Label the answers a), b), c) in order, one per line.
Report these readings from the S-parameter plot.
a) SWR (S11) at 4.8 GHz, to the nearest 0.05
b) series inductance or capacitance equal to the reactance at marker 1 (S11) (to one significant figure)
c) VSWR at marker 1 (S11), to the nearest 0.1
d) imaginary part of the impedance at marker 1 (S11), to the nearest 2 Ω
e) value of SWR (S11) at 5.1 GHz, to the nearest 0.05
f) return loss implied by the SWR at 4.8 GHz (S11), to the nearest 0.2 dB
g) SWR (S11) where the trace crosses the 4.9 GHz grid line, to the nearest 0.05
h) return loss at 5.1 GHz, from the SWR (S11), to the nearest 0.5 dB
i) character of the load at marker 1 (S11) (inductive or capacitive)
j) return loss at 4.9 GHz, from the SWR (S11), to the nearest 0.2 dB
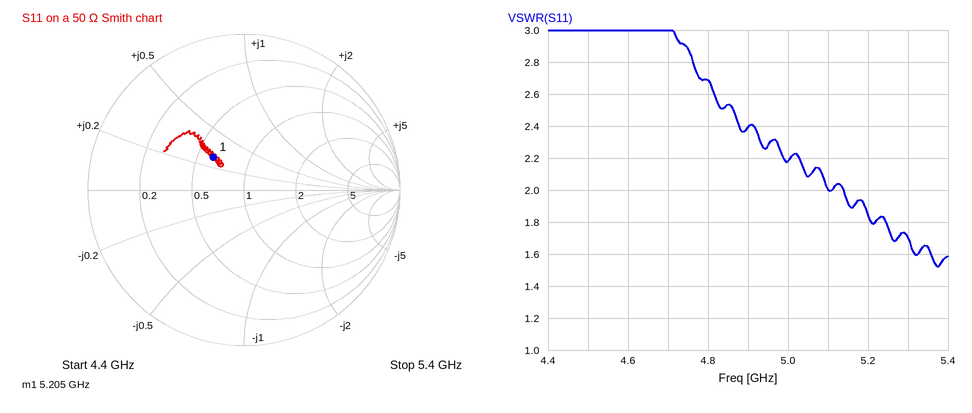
a) 2.70
b) 400 pH
c) 1.8
d) +14 Ω
e) 2.00
f) 6.8 dB
g) 2.40
h) 9.5 dB
i) inductive
j) 7.8 dB
